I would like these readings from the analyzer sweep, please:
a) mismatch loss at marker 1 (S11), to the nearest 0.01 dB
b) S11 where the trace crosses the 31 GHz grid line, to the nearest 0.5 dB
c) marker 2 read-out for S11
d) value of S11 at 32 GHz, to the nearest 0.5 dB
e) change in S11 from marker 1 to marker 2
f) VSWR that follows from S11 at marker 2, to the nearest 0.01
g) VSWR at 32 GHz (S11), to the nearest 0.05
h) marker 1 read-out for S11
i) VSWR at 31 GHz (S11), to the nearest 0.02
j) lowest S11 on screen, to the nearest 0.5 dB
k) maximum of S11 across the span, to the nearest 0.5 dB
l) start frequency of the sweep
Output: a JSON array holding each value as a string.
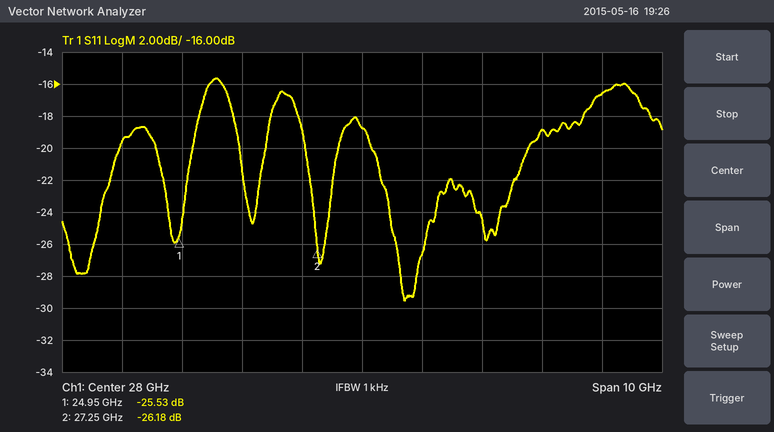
["0.01 dB", "-19.0 dB", "-26.18 dB", "-16.5 dB", "-0.65 dB", "1.10", "1.35", "-25.53 dB", "1.26", "-29.5 dB", "-15.5 dB", "23 GHz"]
